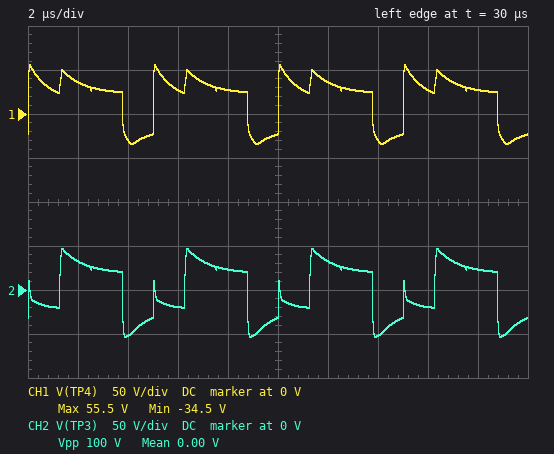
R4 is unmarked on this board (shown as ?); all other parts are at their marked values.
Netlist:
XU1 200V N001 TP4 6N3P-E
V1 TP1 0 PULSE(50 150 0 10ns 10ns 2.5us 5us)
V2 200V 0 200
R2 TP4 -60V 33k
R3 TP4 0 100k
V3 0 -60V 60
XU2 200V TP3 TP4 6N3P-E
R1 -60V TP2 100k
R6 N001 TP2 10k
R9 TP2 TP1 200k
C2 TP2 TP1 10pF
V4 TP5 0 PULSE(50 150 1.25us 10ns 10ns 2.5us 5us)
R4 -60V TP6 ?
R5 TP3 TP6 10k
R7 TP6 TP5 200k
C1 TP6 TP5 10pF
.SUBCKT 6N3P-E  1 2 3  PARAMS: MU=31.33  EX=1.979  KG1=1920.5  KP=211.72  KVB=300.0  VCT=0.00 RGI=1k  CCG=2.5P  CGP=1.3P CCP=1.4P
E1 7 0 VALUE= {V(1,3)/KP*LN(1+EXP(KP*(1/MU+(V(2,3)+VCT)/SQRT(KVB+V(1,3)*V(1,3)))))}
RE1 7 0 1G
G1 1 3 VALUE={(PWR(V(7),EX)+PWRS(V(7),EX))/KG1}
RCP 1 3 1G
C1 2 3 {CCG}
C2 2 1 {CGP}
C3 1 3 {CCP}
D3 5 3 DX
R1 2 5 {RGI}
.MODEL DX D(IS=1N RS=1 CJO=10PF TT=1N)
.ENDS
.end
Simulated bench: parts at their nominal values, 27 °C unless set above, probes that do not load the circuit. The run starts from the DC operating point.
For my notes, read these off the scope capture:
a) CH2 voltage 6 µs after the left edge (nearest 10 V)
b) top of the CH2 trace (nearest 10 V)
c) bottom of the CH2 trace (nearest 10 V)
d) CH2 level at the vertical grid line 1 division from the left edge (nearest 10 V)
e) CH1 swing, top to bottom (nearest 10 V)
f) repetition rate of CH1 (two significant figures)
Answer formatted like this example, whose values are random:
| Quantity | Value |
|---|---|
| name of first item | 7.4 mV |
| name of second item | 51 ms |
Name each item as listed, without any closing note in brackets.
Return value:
| Quantity | Value |
|---|---|
| CH2 voltage 6 µs after the left edge | -20 V |
| top of the CH2 trace | 50 V |
| bottom of the CH2 trace | -50 V |
| CH2 level at the vertical grid line 1 division from the left edge | 30 V |
| CH1 swing, top to bottom | 90 V |
| repetition rate of CH1 | 200 kHz |
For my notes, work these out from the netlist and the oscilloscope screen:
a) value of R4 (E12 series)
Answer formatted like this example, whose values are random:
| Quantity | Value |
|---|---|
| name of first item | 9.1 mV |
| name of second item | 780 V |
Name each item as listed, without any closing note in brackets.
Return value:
| Quantity | Value |
|---|---|
| value of R4 | 120 kΩ |
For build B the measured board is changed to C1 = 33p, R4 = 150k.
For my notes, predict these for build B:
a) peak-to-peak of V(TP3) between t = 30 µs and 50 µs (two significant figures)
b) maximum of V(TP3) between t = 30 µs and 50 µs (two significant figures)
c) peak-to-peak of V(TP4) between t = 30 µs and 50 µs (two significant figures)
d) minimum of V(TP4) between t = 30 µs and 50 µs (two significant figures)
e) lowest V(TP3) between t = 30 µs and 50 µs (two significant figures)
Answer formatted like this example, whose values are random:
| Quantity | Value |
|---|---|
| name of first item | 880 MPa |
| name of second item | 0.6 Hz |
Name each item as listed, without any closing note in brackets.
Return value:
| Quantity | Value |
|---|---|
| peak-to-peak of V(TP3) between t = 30 µs and 50 µs | 110 V |
| maximum of V(TP3) between t = 30 µs and 50 µs | 62 V |
| peak-to-peak of V(TP4) between t = 30 µs and 50 µs | 100 V |
| minimum of V(TP4) between t = 30 µs and 50 µs | -36 V |
| lowest V(TP3) between t = 30 µs and 50 µs | -49 V |
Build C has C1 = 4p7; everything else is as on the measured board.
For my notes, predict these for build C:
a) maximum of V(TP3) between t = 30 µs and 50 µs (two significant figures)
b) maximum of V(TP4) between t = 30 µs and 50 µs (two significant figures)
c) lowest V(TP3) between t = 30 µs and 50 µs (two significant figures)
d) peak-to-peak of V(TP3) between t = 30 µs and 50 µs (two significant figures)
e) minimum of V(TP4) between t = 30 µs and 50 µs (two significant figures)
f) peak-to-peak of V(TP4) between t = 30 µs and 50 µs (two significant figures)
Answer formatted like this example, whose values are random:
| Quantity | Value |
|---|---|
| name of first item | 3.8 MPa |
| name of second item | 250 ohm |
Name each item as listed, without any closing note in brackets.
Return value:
| Quantity | Value |
|---|---|
| maximum of V(TP3) between t = 30 µs and 50 µs | 25 V |
| maximum of V(TP4) between t = 30 µs and 50 µs | 54 V |
| lowest V(TP3) between t = 30 µs and 50 µs | -41 V |
| peak-to-peak of V(TP3) between t = 30 µs and 50 µs | 66 V |
| minimum of V(TP4) between t = 30 µs and 50 µs | -32 V |
| peak-to-peak of V(TP4) between t = 30 µs and 50 µs | 86 V |
